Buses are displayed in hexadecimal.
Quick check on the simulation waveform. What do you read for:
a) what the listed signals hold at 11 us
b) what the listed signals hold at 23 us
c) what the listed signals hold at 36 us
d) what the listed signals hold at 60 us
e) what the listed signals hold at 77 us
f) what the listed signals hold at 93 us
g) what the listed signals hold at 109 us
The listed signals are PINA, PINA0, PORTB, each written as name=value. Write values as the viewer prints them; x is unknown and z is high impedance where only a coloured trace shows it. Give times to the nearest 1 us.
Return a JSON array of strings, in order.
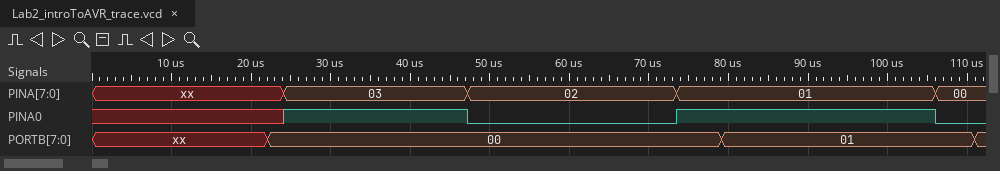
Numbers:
["PINA=xx, PINA0=x, PORTB=xx", "PINA=xx, PINA0=x, PORTB=00", "PINA=03, PINA0=1, PORTB=00", "PINA=02, PINA0=0, PORTB=00", "PINA=01, PINA0=1, PORTB=00", "PINA=01, PINA0=1, PORTB=01", "PINA=00, PINA0=0, PORTB=01"]
